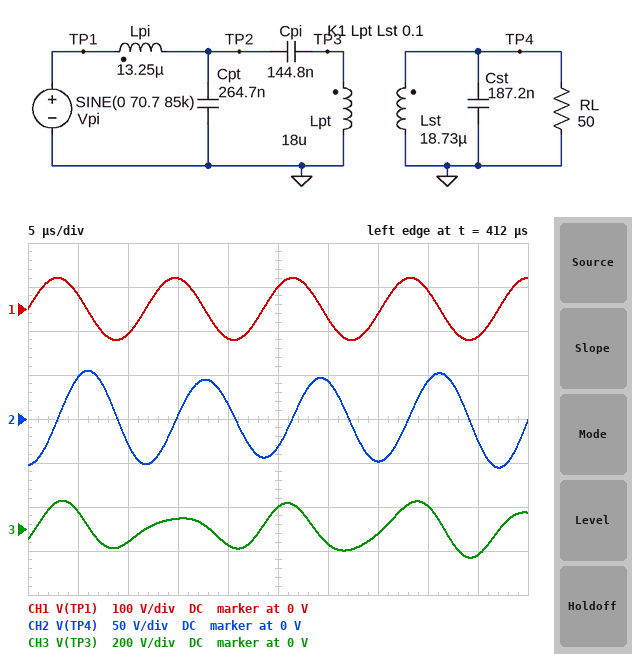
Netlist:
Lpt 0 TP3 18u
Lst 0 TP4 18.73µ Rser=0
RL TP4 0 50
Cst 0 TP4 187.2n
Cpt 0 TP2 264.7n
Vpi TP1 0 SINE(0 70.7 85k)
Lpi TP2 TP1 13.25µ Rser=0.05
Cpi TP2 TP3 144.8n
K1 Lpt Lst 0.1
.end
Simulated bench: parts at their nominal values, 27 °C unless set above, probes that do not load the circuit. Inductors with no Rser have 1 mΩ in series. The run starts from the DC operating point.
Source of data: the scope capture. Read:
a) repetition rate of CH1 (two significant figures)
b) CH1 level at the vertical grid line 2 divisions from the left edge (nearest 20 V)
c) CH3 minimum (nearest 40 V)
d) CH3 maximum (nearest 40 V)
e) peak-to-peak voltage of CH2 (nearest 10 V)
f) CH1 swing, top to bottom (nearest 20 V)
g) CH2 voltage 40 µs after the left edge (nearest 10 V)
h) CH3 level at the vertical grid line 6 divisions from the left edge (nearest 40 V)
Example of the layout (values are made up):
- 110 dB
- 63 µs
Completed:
- 85 kHz
- -60 V
- -120 V
- 120 V
- 110 V
- 140 V
- 40 V
- -80 V
